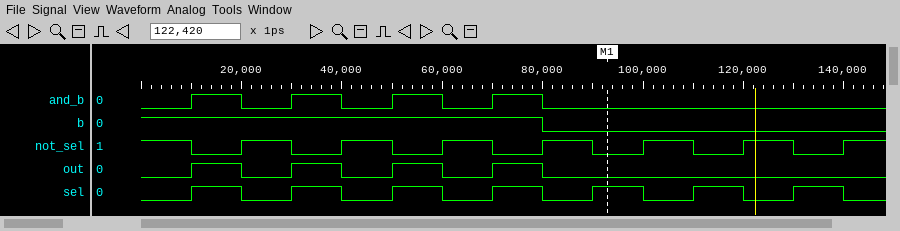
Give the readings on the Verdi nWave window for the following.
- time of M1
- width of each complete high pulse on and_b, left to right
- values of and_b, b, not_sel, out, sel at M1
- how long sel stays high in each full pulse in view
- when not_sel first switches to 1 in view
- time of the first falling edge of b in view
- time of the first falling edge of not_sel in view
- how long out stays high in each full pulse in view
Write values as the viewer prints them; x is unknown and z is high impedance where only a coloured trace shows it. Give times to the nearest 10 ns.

90 ns
10 ns, 10 ns, 10 ns, 10 ns
and_b=0, b=0, not_sel=0, out=0, sel=1
10 ns, 10 ns, 10 ns, 10 ns, 10 ns, 10 ns, 10 ns
20 ns
80 ns
10 ns
10 ns, 10 ns, 10 ns, 10 ns
